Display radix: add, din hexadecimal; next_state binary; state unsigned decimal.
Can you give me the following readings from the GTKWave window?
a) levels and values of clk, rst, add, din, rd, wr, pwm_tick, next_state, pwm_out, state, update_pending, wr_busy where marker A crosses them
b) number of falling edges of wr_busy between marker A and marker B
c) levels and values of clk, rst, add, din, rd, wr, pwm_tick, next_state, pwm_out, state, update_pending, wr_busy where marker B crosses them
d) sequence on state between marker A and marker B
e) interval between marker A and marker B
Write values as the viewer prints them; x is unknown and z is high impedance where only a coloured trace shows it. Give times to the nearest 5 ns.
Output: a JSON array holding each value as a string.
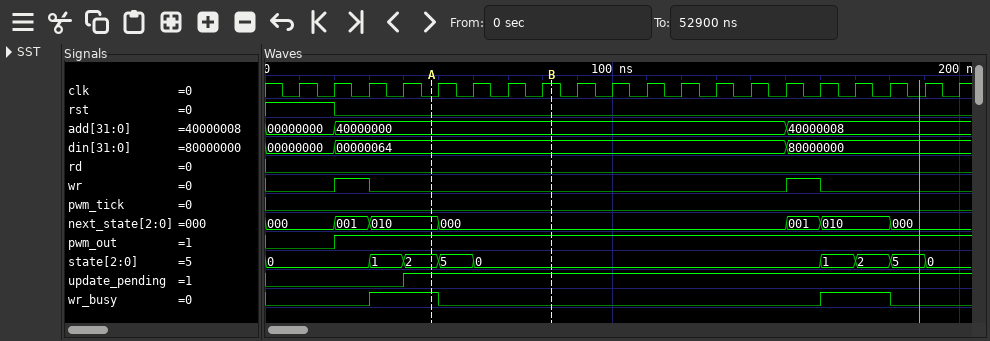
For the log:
["clk=0, rst=0, add=40000000, din=00000064, rd=0, wr=0, pwm_tick=0, next_state=010, pwm_out=1, state=2, update_pending=1, wr_busy=1", "1", "clk=1, rst=0, add=40000000, din=00000064, rd=0, wr=0, pwm_tick=0, next_state=000, pwm_out=1, state=0, update_pending=1, wr_busy=0", "2, 5, 0", "35 ns"]
